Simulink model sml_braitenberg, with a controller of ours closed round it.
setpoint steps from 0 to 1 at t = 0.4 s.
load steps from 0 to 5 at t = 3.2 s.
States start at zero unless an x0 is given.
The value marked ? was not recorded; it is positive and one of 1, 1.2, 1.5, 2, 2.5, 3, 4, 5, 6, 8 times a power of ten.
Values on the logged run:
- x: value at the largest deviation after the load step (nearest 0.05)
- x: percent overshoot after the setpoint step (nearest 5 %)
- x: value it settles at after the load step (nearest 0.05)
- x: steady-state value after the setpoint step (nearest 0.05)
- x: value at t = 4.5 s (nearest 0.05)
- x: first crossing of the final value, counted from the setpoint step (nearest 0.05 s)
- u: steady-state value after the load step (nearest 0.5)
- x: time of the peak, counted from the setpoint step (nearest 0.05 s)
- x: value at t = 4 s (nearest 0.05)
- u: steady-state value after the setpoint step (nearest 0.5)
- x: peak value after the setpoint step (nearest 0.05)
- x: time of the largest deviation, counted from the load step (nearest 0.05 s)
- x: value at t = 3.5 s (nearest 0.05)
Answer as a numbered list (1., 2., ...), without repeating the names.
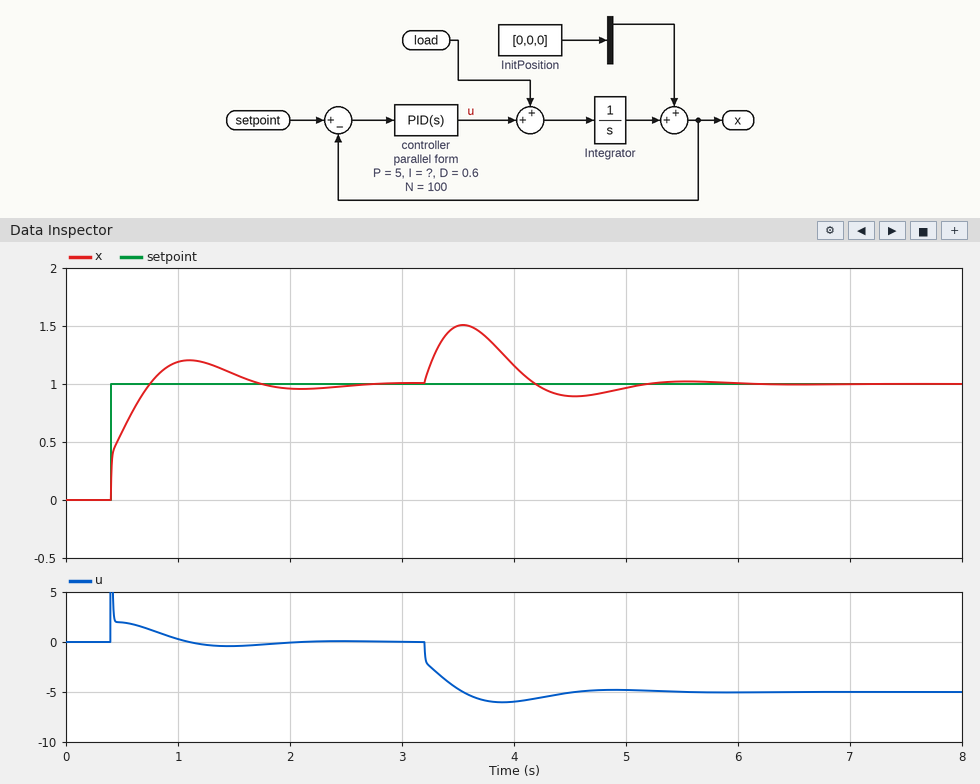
1. 1.50
2. 20 %
3. 1.00
4. 1.00
5. 0.90
6. 0.35 s
7. -5.0
8. 0.70 s
9. 1.15
10. 0.0
11. 1.20
12. 0.35 s
13. 1.50
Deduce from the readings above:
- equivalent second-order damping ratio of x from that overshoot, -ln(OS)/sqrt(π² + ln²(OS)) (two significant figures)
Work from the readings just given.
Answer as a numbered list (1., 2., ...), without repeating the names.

1. 0.46
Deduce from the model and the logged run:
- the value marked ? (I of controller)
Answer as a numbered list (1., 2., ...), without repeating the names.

1. 20
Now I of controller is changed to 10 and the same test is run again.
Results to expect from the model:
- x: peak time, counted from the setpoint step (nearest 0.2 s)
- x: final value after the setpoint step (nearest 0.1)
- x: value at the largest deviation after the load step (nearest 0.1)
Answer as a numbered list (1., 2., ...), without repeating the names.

1. 1.0 s
2. 1.0
3. 1.6
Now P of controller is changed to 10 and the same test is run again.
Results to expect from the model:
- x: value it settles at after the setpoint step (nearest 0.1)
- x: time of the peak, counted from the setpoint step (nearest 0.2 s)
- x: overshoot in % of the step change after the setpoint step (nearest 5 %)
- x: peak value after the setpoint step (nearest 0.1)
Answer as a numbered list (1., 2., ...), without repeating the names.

1. 1.0
2. 0.6 s
3. 10 %
4. 1.1
